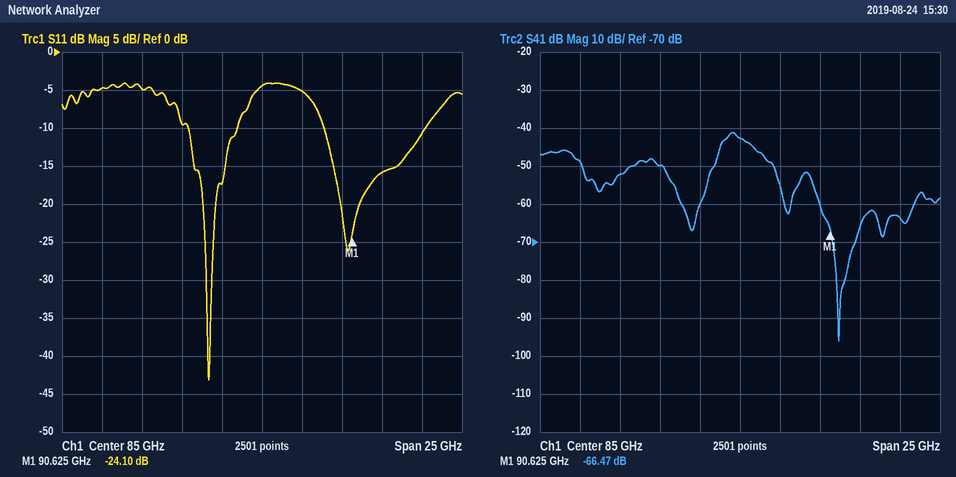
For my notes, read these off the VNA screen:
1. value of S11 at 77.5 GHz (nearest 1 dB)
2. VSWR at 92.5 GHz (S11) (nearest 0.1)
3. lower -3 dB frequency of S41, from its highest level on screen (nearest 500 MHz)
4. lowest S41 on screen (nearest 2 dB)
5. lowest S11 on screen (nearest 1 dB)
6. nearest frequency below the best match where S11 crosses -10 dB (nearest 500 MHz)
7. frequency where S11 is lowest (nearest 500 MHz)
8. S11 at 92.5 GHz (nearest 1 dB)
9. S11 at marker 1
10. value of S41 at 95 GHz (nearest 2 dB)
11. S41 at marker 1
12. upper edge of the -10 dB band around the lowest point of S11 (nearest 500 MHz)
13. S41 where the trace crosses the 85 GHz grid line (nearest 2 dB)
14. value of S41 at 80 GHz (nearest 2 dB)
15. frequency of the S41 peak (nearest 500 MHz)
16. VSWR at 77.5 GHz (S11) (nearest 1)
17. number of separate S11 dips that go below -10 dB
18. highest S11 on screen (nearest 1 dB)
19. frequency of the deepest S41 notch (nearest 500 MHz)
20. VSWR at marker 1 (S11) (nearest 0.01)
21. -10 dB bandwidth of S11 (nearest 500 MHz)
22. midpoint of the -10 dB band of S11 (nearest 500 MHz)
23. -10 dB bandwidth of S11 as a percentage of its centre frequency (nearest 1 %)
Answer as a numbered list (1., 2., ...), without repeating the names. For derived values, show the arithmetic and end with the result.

1. -5 dB
2. |Γ| = 10^(-16/20) = 0.1585; VSWR = (1 + 0.1585)/(1 − 0.1585) ≈ 1.4
3. 84.0 GHz
4. -96 dB
5. -43 dB
6. 80.5 GHz
7. 81.5 GHz
8. -16 dB
9. -24.10 dB
10. -64 dB
11. -66.47 dB
12. 83.5 GHz
13. -42 dB
14. -50 dB
15. 84.5 GHz
16. |Γ| = 10^(-5/20) = 0.5623; VSWR = (1 + 0.5623)/(1 − 0.5623) ≈ 4
17. 2
18. -4 dB
19. 91.0 GHz
20. (1 + 0.0624)/(1 − 0.0624) ≈ 1.13
21. 83.5 GHz − 80.5 GHz = 3.0 GHz
22. 82.0 GHz
23. 3 GHz / 82 GHz ≈ 4 %
